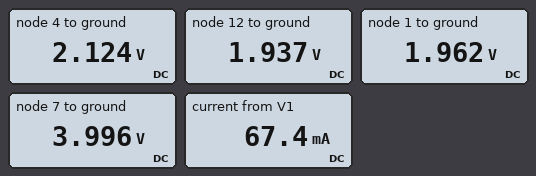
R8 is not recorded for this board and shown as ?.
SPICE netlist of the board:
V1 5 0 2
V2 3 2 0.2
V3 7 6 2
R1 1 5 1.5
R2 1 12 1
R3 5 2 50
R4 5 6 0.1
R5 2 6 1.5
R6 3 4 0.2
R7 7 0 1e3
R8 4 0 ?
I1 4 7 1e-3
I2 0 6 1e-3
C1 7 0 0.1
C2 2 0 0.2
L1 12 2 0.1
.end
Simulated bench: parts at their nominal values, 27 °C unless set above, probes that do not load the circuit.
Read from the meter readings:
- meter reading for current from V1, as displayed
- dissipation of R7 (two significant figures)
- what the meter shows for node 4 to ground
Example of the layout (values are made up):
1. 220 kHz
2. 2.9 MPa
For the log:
1. 67.4 mA
2. 16 mW
3. 2.124 V
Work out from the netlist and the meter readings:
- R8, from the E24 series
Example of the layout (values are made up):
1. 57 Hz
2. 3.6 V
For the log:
1. 33 Ω
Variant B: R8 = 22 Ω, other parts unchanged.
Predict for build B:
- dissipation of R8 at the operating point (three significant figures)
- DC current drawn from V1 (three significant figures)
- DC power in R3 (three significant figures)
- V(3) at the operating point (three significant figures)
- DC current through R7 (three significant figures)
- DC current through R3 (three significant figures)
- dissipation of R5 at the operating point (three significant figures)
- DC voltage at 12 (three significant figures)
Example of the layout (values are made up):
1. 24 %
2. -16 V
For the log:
1. 198 mW
2. 97.9 mA
3. 169 µW
4. 2.11 V
5. 3.99 mA
6. 1.84 mA
7. 4.93 mW
8. 1.91 V
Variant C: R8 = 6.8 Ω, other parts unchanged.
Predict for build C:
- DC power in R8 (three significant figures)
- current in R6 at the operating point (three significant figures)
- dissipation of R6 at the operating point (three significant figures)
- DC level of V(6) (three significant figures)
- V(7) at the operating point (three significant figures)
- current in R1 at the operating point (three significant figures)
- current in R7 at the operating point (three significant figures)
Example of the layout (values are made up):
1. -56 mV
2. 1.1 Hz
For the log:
1. 519 mW
2. 277 mA
3. 15.4 mW
4. 1.98 V
5. 3.98 V
6. 106 mA
7. 3.98 mA
